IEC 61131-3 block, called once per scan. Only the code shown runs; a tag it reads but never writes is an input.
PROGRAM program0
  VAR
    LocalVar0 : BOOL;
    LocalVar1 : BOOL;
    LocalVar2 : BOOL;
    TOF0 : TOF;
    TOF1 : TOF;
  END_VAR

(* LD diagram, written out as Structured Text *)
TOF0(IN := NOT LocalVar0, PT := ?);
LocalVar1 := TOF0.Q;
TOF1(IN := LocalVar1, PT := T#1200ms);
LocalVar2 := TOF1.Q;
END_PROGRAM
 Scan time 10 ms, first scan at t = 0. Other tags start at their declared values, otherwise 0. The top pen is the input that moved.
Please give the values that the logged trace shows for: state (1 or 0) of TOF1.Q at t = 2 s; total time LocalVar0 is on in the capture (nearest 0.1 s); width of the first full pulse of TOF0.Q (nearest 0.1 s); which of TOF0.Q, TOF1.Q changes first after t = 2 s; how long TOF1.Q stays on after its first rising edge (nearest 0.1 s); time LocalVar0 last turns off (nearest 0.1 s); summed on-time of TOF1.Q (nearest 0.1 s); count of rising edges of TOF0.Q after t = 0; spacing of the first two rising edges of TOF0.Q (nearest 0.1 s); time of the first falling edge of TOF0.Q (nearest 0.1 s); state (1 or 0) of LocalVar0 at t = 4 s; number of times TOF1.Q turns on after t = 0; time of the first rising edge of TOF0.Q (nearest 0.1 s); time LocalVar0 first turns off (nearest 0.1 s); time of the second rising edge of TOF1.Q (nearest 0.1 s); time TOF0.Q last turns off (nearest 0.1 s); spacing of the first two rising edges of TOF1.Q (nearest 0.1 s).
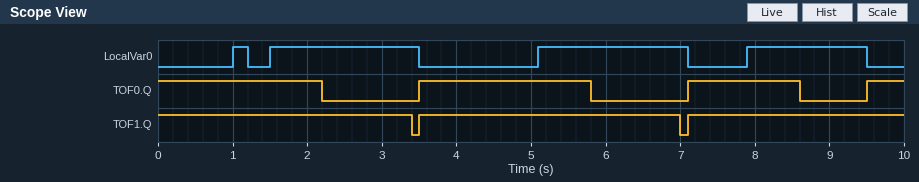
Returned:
1
5.8 s
2.3 s
TOF0.Q
3.5 s
9.5 s
9.8 s
3
3.6 s
2.2 s
0
2
3.5 s
1.2 s
7.1 s
8.6 s
3.6 s
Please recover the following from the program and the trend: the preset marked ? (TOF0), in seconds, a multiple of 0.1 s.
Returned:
0.7 s
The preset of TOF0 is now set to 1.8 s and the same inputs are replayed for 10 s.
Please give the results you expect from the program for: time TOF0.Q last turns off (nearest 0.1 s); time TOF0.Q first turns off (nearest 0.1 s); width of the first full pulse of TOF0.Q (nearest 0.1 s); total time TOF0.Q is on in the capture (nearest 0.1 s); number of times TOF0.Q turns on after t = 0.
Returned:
6.9 s
3.3 s
3.4 s
9.6 s
2
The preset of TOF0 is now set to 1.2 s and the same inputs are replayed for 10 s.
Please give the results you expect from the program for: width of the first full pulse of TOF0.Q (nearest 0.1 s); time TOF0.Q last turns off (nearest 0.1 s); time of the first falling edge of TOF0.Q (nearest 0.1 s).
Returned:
2.8 s
9.1 s
2.7 s
